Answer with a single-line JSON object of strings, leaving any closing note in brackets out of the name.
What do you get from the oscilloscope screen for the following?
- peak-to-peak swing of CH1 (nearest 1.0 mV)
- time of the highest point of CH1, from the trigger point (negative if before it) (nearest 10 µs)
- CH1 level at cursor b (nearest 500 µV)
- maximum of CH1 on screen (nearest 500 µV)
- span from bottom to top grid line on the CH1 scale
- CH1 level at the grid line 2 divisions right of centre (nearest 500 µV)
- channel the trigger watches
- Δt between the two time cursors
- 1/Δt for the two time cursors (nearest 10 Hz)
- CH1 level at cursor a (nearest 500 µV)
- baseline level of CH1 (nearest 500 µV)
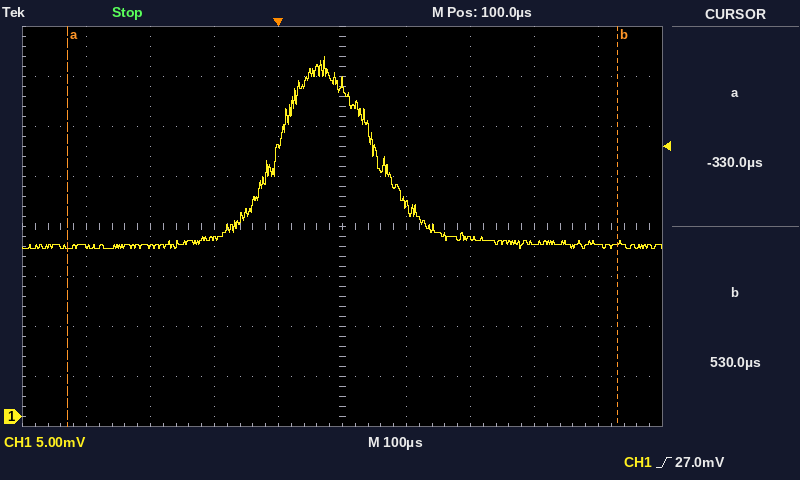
{"peak-to-peak swing of CH1": "19.0 mV", "time of the highest point of CH1, from the trigger point (negative if before it)": "+70 µs", "CH1 level at cursor b": "17.5 mV", "maximum of CH1 on screen": "36.0 mV", "span from bottom to top grid line on the CH1 scale": "40 mV", "CH1 level at the grid line 2 divisions right of centre": "18.0 mV", "channel the trigger watches": "CH1", "Δt between the two time cursors": "860 µs", "1/Δt for the two time cursors": "1.16 kHz", "CH1 level at cursor a": "17.0 mV", "baseline level of CH1": "17.0 mV"}
